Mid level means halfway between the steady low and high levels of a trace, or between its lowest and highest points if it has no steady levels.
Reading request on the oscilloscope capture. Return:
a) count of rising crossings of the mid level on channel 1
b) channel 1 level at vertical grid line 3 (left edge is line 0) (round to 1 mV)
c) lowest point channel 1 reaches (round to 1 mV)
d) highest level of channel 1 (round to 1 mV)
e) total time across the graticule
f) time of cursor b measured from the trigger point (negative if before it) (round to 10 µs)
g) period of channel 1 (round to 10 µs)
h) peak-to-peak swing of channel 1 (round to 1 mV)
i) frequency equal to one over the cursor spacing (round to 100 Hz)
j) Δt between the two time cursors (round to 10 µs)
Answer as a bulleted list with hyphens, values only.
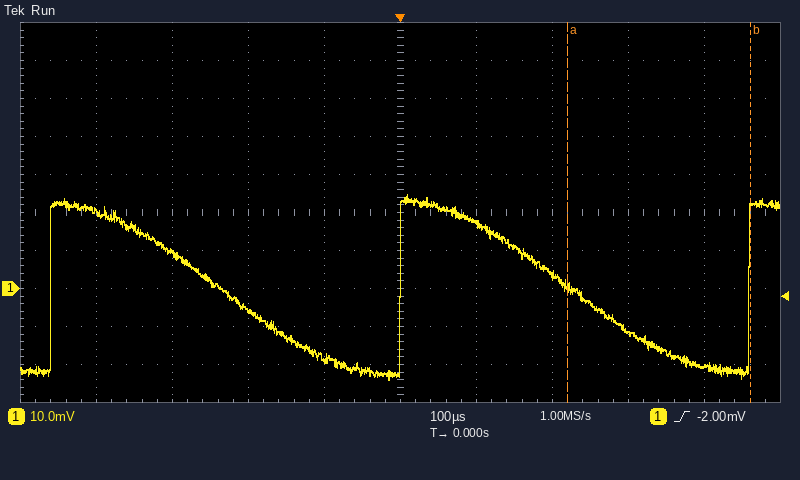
- 3
- -6 mV
- -24 mV
- 25 mV
- 1 ms
- +460 µs
- 460 µs
- 49 mV
- 4.2 kHz
- 240 µs
